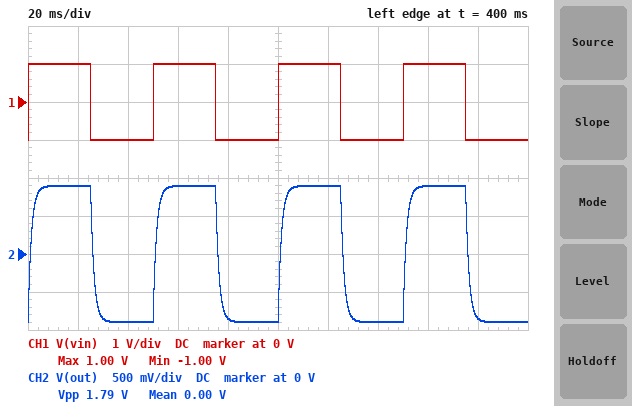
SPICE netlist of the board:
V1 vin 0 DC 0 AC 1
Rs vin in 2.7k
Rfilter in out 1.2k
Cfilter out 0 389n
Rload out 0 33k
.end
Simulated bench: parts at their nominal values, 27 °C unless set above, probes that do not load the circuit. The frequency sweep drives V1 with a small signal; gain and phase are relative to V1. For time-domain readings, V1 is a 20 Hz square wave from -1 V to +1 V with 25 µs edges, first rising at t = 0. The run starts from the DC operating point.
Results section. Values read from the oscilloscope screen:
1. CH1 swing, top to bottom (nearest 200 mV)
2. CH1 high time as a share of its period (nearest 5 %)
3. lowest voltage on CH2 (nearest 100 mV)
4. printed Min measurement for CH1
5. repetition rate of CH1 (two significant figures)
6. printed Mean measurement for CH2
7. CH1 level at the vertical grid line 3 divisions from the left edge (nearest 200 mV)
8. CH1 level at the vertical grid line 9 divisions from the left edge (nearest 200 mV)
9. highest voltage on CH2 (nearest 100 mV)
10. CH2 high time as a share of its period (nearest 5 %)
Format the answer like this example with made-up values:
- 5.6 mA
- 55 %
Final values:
- 2.0 V
- 50 %
- -900 mV
- -1.00 V
- 20 Hz
- 0.00 V
- 1.0 V
- -1.0 V
- 900 mV
- 50 %
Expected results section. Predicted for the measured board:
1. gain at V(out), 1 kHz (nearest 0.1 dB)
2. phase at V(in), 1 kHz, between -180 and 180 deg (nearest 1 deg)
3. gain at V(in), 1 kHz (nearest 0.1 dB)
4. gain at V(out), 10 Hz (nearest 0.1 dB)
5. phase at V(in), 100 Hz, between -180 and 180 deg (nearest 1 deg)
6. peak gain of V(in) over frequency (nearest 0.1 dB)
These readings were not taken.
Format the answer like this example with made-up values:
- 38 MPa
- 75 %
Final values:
- -19.6 dB
- -13 deg
- -9.8 dB
- -1.0 dB
- -25 deg
- -0.7 dB
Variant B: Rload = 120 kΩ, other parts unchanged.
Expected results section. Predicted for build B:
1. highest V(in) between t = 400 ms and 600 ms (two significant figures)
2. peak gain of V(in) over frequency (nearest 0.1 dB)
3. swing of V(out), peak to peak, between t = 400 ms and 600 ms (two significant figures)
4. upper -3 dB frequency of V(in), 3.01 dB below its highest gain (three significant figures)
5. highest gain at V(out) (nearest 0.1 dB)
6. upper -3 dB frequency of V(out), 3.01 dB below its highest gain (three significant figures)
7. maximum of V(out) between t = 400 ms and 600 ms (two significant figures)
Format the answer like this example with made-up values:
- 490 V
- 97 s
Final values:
- 980 mV
- -0.2 dB
- 1.9 V
- 121 Hz
- -0.3 dB
- 108 Hz
- 970 mV
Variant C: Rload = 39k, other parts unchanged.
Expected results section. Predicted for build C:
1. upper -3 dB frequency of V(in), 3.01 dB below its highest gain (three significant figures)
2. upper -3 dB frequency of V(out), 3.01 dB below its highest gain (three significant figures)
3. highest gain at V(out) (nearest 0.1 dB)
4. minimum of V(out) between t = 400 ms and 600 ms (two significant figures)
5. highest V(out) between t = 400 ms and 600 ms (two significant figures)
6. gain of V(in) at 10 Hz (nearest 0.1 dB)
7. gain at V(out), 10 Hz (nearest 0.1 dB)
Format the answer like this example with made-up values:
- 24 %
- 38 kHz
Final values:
- 130 Hz
- 115 Hz
- -0.8 dB
- -910 mV
- 910 mV
- -0.6 dB
- -0.9 dB
